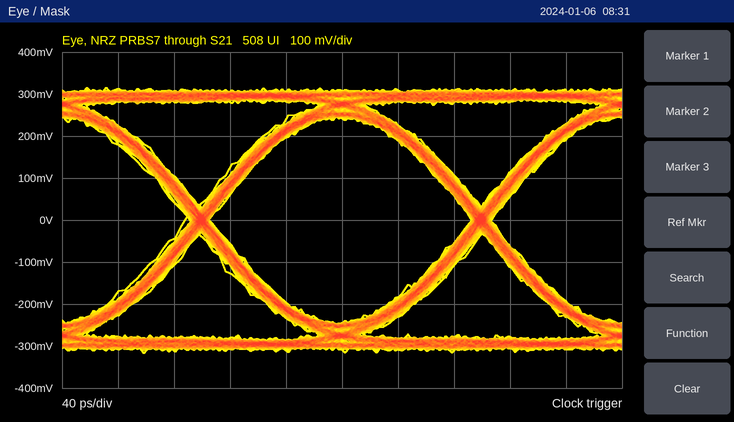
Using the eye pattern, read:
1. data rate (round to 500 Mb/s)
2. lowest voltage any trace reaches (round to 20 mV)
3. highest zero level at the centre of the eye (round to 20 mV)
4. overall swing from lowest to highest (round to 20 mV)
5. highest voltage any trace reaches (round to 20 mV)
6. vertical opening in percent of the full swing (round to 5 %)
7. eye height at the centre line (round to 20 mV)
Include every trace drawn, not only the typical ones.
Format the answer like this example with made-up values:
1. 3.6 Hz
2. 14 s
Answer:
1. 5.0 Gb/s
2. -320 mV
3. -240 mV
4. 640 mV
5. 320 mV
6. 75 %
7. 480 mV
